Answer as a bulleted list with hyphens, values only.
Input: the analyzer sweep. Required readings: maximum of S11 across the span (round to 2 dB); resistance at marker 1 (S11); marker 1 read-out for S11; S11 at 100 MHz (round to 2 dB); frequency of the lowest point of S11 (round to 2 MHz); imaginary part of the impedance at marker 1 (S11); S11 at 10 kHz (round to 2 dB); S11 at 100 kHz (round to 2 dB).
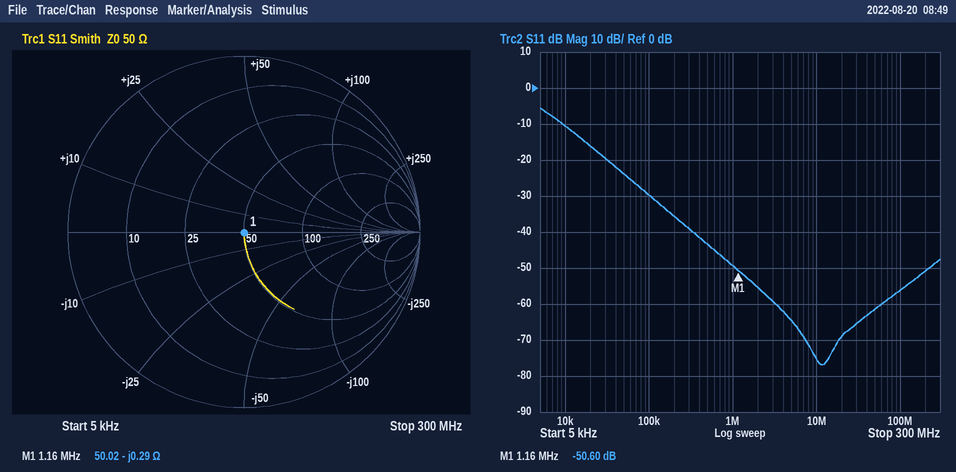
- -6 dB
- 50.02 Ω
- -50.60 dB
- -56 dB
- 12 MHz
- -0.29 Ω
- -10 dB
- -30 dB
